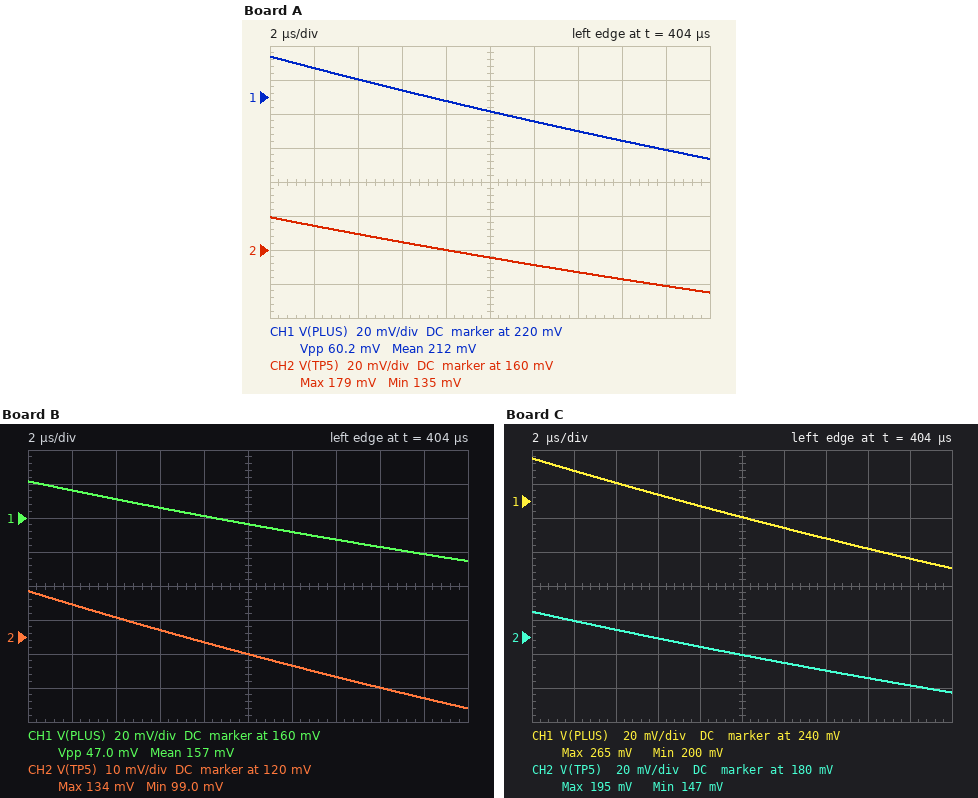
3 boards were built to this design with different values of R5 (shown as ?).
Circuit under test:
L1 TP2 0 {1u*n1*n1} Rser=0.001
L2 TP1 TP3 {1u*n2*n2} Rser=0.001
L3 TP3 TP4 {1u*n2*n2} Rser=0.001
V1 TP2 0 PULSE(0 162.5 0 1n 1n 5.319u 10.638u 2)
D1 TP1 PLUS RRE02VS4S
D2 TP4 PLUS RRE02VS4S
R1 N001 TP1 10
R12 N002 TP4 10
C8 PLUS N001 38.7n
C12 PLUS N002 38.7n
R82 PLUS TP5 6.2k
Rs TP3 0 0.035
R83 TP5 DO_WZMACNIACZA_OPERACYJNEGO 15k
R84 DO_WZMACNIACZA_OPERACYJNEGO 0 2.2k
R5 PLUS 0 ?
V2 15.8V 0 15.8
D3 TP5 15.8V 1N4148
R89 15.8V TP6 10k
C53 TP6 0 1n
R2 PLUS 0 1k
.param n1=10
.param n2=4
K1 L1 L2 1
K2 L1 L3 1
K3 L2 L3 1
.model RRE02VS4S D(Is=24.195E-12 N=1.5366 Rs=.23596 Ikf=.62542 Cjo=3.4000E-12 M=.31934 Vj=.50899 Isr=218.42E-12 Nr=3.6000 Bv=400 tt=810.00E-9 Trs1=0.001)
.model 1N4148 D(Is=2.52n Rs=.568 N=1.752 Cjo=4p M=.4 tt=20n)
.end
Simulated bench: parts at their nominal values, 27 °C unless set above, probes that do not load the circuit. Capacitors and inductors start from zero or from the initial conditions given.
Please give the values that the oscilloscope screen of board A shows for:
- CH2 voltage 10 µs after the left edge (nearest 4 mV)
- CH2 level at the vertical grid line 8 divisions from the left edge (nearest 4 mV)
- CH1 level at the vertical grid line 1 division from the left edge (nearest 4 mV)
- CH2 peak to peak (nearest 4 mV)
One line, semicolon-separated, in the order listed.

156 mV; 144 mV; 236 mV; 44 mV
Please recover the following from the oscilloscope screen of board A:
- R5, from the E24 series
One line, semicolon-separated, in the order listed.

16 kΩ
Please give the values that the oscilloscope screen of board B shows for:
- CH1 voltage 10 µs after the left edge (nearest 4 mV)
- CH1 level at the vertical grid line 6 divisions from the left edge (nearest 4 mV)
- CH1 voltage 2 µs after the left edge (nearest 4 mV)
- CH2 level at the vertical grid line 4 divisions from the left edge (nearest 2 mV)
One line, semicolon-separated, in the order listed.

156 mV; 152 mV; 176 mV; 118 mV
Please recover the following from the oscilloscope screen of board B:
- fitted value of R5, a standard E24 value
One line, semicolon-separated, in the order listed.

8.2 kΩ
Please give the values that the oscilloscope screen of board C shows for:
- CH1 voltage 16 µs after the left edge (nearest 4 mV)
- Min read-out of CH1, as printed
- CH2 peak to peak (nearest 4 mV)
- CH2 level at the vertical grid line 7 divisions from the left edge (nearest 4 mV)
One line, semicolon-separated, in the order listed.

212 mV; 200 mV; 48 mV; 160 mV
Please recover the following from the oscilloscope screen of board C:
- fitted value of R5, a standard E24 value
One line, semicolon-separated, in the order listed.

22 kΩ
